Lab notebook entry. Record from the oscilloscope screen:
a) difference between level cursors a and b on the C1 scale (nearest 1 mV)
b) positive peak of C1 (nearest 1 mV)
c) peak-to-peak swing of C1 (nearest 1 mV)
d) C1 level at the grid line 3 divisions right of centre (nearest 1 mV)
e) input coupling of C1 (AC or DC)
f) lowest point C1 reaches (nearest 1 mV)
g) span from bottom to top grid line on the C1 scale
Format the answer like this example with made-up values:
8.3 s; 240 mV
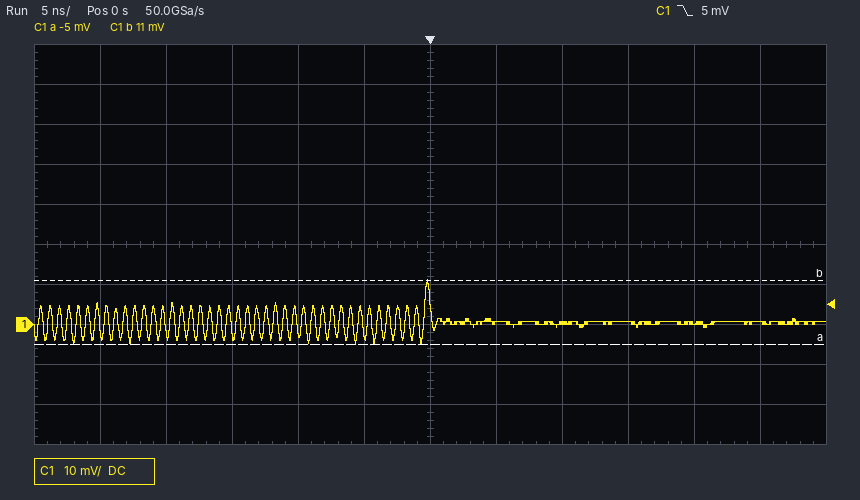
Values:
16 mV; 11 mV; 16 mV; 1 mV; DC; -5 mV; 100 mV
